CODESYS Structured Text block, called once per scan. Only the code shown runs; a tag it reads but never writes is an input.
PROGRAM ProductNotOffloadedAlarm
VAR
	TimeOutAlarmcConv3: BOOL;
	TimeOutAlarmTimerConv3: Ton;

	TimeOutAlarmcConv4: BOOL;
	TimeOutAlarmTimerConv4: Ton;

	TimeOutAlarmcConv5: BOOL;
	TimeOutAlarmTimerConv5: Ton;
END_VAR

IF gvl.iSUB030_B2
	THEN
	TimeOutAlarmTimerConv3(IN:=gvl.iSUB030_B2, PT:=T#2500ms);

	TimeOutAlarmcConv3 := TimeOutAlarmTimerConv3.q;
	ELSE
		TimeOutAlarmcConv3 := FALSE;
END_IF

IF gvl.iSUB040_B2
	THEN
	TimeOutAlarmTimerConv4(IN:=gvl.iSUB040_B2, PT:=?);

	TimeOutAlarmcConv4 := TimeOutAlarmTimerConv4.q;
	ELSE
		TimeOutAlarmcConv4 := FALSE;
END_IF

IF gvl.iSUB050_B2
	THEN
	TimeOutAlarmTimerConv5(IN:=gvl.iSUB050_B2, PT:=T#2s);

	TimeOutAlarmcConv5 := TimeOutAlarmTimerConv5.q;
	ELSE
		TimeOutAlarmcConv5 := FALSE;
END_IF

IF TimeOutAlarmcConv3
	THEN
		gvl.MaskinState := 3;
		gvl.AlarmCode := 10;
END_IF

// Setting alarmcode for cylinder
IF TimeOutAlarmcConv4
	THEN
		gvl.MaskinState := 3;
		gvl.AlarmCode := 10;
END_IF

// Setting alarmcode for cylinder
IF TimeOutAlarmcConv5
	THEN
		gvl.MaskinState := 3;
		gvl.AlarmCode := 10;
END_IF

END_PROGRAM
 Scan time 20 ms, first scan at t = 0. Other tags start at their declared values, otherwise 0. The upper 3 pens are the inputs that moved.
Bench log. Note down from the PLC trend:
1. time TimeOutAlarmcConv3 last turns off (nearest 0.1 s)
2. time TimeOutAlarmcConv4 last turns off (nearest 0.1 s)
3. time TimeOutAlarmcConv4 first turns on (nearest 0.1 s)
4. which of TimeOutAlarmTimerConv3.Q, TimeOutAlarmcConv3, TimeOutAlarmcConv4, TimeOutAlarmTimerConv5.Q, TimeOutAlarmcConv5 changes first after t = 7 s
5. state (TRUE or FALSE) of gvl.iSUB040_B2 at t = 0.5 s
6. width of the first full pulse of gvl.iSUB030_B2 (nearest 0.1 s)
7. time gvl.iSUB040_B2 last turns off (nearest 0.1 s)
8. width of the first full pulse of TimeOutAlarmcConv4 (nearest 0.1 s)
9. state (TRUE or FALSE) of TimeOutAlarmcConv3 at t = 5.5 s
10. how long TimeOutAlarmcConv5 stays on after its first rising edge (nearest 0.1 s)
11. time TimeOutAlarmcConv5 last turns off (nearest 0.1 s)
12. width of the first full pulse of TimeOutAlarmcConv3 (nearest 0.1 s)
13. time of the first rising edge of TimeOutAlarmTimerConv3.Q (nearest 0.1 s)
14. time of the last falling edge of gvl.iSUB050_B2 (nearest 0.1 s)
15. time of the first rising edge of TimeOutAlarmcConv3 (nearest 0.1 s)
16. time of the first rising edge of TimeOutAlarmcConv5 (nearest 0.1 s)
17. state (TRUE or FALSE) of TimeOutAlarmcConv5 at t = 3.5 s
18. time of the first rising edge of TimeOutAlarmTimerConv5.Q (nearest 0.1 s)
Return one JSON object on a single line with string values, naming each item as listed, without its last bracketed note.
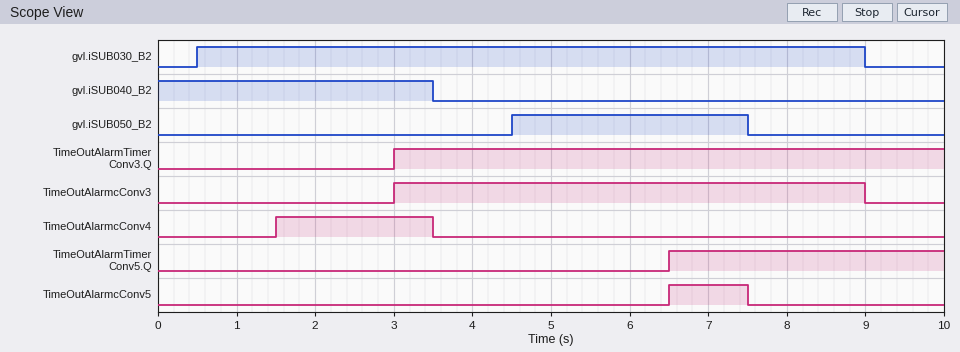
{"time TimeOutAlarmcConv3 last turns off": "9.0 s", "time TimeOutAlarmcConv4 last turns off": "3.5 s", "time TimeOutAlarmcConv4 first turns on": "1.5 s", "which of TimeOutAlarmTimerConv3.Q, TimeOutAlarmcConv3, TimeOutAlarmcConv4, TimeOutAlarmTimerConv5.Q, TimeOutAlarmcConv5 changes first after t = 7 s": "TimeOutAlarmcConv5", "state (TRUE or FALSE) of gvl.iSUB040_B2 at t = 0.5 s": "TRUE", "width of the first full pulse of gvl.iSUB030_B2": "8.5 s", "time gvl.iSUB040_B2 last turns off": "3.5 s", "width of the first full pulse of TimeOutAlarmcConv4": "2.0 s", "state (TRUE or FALSE) of TimeOutAlarmcConv3 at t = 5.5 s": "TRUE", "how long TimeOutAlarmcConv5 stays on after its first rising edge": "1.0 s", "time TimeOutAlarmcConv5 last turns off": "7.5 s", "width of the first full pulse of TimeOutAlarmcConv3": "6.0 s", "time of the first rising edge of TimeOutAlarmTimerConv3.Q": "3.0 s", "time of the last falling edge of gvl.iSUB050_B2": "7.5 s", "time of the first rising edge of TimeOutAlarmcConv3": "3.0 s", "time of the first rising edge of TimeOutAlarmcConv5": "6.5 s", "state (TRUE or FALSE) of TimeOutAlarmcConv5 at t = 3.5 s": "FALSE", "time of the first rising edge of TimeOutAlarmTimerConv5.Q": "6.5 s"}
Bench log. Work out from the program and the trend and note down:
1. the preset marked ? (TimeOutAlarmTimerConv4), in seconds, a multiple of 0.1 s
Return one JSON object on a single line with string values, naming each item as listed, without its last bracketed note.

{"the preset marked ? (TimeOutAlarmTimerConv4), in seconds, a multiple of 0.1 s": "1.5 s"}
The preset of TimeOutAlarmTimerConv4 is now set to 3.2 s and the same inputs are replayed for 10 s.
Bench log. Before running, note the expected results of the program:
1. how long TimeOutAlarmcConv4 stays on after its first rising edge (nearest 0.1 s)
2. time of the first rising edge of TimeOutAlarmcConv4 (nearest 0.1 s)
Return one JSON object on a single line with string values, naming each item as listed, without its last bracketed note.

{"how long TimeOutAlarmcConv4 stays on after its first rising edge": "0.3 s", "time of the first rising edge of TimeOutAlarmcConv4": "3.2 s"}
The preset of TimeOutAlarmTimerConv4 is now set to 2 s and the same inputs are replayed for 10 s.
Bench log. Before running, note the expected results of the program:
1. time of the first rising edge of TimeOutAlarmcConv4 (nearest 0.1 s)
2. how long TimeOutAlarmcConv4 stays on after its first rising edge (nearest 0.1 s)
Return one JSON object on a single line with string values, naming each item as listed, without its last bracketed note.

{"time of the first rising edge of TimeOutAlarmcConv4": "2.0 s", "how long TimeOutAlarmcConv4 stays on after its first rising edge": "1.5 s"}
